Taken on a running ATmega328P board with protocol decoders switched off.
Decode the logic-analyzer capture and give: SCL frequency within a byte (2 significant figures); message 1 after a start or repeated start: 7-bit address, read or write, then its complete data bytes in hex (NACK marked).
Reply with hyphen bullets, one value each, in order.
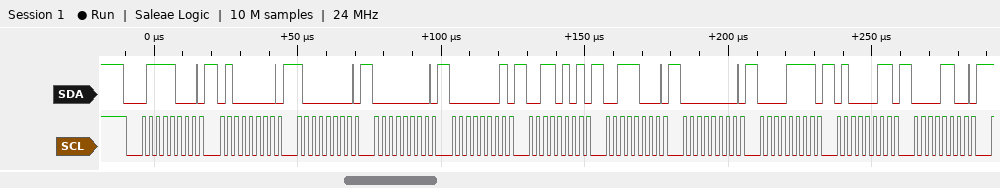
- 400 kHz
- 0x3C write: 40 80 00 01 35 38 00 0F 43 0C
